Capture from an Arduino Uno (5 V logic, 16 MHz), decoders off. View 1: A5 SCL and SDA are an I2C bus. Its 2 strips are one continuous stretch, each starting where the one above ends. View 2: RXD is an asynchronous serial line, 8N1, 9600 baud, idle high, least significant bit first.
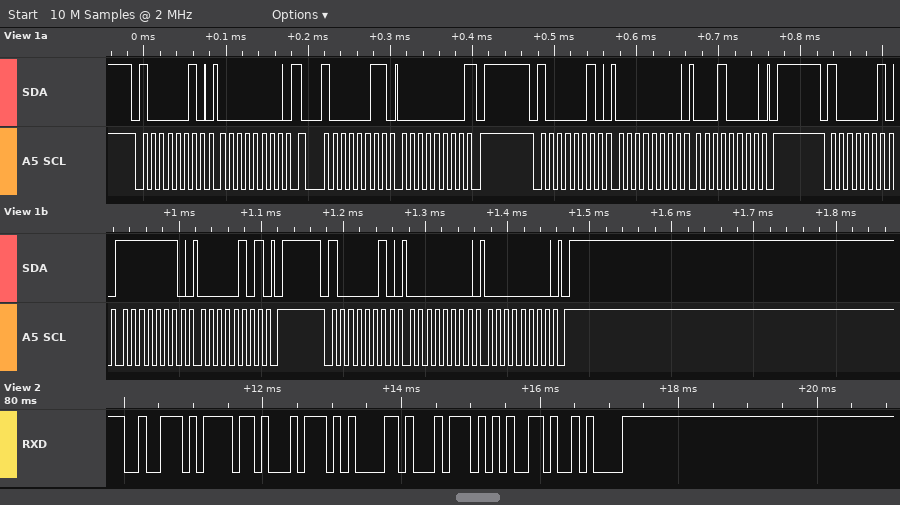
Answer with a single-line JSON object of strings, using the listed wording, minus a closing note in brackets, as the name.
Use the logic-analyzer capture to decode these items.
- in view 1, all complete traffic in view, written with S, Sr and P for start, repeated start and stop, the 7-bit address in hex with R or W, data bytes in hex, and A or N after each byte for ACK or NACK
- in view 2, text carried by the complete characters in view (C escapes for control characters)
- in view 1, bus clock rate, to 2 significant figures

{"in view 1, all complete traffic in view, written with S, Sr and P for start, repeated start and stop, the 7-bit address in hex with R or W, data bytes in hex, and A or N after each byte for ACK or NACK": "S 41W A 00 A Sr 41R A 00 N P S 41W A 00 A 10 A P S 41W A FE A 05 A P S 41W A 00 A 00 A P", "in view 2, text carried by the complete characters in view": "\"rotate\\n\"", "in view 1, bus clock rate, to 2 significant figures": "100 kHz"}
